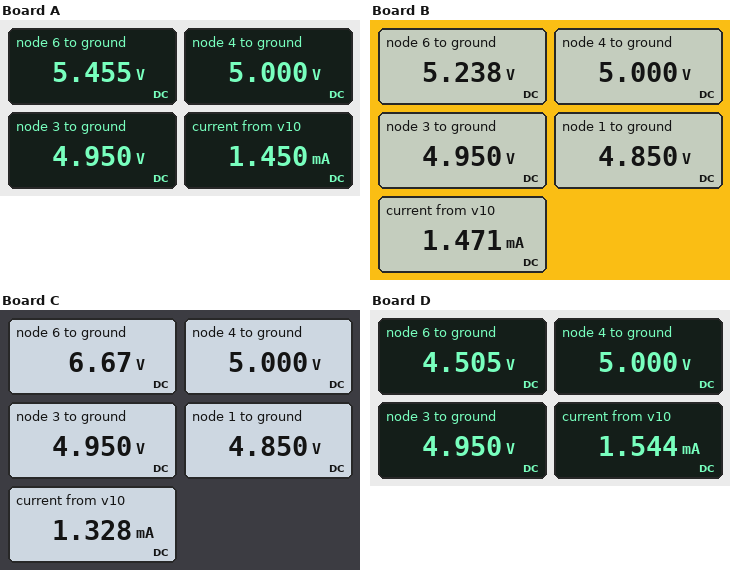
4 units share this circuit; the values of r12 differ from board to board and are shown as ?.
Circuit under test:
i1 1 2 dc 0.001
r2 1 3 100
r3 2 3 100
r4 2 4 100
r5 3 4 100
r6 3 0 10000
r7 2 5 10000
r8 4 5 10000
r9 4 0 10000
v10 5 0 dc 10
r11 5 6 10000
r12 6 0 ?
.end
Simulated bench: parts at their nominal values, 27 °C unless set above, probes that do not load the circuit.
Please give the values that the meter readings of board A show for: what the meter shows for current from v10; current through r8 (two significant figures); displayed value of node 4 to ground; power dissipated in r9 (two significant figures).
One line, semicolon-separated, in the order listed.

1.450 mA; 500 µA; 5.000 V; 2.5 mW
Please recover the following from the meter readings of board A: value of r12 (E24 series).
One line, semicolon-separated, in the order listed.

12 kΩ
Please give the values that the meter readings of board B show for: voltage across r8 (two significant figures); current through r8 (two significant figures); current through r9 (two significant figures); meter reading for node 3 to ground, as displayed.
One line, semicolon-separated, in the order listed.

5.0 V; 500 µA; 500 µA; 4.950 V
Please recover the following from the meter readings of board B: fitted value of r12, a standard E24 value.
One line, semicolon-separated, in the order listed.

11 kΩ
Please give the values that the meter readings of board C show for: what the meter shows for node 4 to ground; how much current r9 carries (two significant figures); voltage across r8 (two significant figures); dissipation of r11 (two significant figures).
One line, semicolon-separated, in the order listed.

5.000 V; 500 µA; 5.0 V; 1.1 mW
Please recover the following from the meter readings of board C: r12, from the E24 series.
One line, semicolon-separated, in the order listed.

20 kΩ
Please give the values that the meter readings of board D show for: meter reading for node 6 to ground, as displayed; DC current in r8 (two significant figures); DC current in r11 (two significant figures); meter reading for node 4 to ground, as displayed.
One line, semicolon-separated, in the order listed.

4.505 V; 500 µA; 550 µA; 5.000 V
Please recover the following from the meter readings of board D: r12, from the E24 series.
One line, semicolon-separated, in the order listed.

8.2 kΩ
